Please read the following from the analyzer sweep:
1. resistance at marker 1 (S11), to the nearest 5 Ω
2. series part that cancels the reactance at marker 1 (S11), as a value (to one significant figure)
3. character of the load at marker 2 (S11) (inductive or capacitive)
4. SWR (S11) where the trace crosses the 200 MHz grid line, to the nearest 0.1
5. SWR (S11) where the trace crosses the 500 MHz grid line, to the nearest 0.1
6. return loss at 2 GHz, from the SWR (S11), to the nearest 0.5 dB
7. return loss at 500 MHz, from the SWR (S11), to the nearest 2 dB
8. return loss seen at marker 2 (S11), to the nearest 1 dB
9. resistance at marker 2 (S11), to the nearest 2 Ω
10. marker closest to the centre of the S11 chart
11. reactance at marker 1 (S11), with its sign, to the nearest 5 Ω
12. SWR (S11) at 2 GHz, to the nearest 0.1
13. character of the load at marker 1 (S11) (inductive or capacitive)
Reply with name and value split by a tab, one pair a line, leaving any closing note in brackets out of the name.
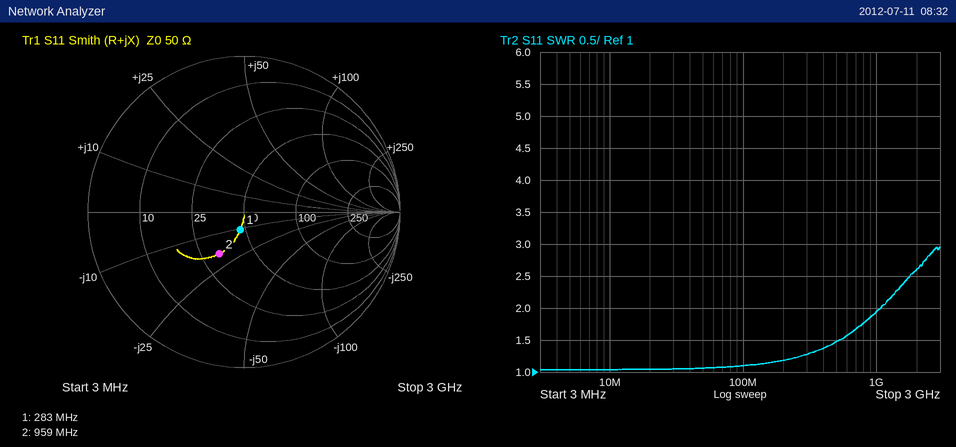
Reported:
resistance at marker 1 (S11), to the nearest 5 Ω	45 Ω
series part that cancels the reactance at marker 1 (S11), as a value	6 nH
character of the load at marker 2 (S11)	capacitive
SWR (S11) where the trace crosses the 200 MHz grid line, to the nearest 0.1	1.2
SWR (S11) where the trace crosses the 500 MHz grid line, to the nearest 0.1	1.5
return loss at 2 GHz, from the SWR (S11), to the nearest 0.5 dB	7.0 dB
return loss at 500 MHz, from the SWR (S11), to the nearest 2 dB	14 dB
return loss seen at marker 2 (S11), to the nearest 1 dB	10 dB
resistance at marker 2 (S11), to the nearest 2 Ω	32 Ω
marker closest to the centre of the S11 chart	marker 1
reactance at marker 1 (S11), with its sign, to the nearest 5 Ω	-10 Ω
SWR (S11) at 2 GHz, to the nearest 0.1	2.6
character of the load at marker 1 (S11)	capacitive
